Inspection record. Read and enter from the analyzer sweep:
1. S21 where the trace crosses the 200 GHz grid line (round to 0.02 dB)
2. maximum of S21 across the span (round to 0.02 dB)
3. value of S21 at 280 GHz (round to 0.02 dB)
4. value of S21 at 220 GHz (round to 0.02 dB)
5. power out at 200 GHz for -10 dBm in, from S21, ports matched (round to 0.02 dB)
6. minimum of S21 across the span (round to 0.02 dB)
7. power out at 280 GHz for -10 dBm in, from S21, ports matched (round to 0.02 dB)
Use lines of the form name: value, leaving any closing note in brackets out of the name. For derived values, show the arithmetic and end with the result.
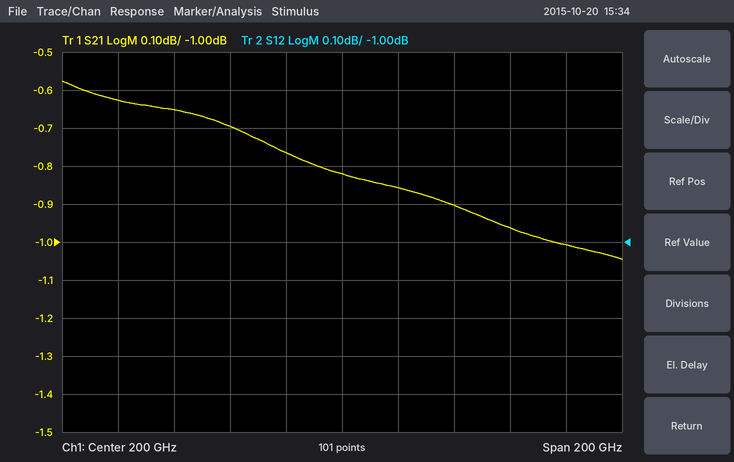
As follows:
S21 where the trace crosses the 200 GHz grid line: -0.82 dB
maximum of S21 across the span: -0.58 dB
value of S21 at 280 GHz: -1.00 dB
value of S21 at 220 GHz: -0.86 dB
power out at 200 GHz for -10 dBm in, from S21, ports matched: -10 dBm + (-0.82 dB) = -10.82 dBm
minimum of S21 across the span: -1.04 dB
power out at 280 GHz for -10 dBm in, from S21, ports matched: -10 dBm + (-1.00 dB) = -11.00 dBm
